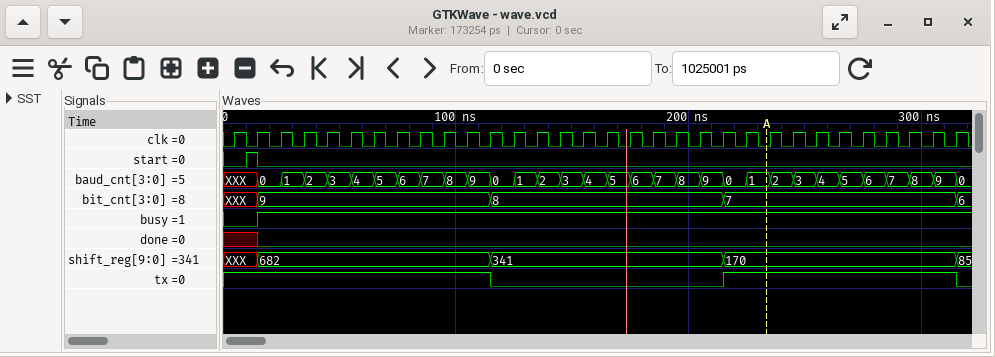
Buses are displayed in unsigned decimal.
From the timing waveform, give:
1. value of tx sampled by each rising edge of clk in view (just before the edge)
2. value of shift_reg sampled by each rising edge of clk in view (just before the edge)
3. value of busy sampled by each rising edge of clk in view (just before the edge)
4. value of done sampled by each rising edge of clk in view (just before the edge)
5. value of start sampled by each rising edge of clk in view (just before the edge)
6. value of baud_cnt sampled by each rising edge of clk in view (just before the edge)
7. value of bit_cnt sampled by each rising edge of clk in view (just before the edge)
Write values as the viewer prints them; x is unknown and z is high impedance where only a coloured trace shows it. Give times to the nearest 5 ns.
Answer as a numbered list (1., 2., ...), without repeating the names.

1. 1 1 1 1 1 1 1 1 1 1 1 1 0 0 0 0 0 0 0 0 0 0 1 1 1 1 1 1 1 1 1 1
2. XXX, XXX, 682, 682, 682, 682, 682, 682, 682, 682, 682, 682, 341, 341, 341, 341, 341, 341, 341, 341, 341, 341, 170, 170, 170, 170, 170, 170, 170, 170, 170, 170
3. 0 0 1 1 1 1 1 1 1 1 1 1 1 1 1 1 1 1 1 1 1 1 1 1 1 1 1 1 1 1 1 1
4. x x 0 0 0 0 0 0 0 0 0 0 0 0 0 0 0 0 0 0 0 0 0 0 0 0 0 0 0 0 0 0
5. 0 1 0 0 0 0 0 0 0 0 0 0 0 0 0 0 0 0 0 0 0 0 0 0 0 0 0 0 0 0 0 0
6. XXX, XXX, 0, 1, 2, 3, 4, 5, 6, 7, 8, 9, 0, 1, 2, 3, 4, 5, 6, 7, 8, 9, 0, 1, 2, 3, 4, 5, 6, 7, 8, 9
7. XXX, XXX, 9, 9, 9, 9, 9, 9, 9, 9, 9, 9, 8, 8, 8, 8, 8, 8, 8, 8, 8, 8, 7, 7, 7, 7, 7, 7, 7, 7, 7, 7
